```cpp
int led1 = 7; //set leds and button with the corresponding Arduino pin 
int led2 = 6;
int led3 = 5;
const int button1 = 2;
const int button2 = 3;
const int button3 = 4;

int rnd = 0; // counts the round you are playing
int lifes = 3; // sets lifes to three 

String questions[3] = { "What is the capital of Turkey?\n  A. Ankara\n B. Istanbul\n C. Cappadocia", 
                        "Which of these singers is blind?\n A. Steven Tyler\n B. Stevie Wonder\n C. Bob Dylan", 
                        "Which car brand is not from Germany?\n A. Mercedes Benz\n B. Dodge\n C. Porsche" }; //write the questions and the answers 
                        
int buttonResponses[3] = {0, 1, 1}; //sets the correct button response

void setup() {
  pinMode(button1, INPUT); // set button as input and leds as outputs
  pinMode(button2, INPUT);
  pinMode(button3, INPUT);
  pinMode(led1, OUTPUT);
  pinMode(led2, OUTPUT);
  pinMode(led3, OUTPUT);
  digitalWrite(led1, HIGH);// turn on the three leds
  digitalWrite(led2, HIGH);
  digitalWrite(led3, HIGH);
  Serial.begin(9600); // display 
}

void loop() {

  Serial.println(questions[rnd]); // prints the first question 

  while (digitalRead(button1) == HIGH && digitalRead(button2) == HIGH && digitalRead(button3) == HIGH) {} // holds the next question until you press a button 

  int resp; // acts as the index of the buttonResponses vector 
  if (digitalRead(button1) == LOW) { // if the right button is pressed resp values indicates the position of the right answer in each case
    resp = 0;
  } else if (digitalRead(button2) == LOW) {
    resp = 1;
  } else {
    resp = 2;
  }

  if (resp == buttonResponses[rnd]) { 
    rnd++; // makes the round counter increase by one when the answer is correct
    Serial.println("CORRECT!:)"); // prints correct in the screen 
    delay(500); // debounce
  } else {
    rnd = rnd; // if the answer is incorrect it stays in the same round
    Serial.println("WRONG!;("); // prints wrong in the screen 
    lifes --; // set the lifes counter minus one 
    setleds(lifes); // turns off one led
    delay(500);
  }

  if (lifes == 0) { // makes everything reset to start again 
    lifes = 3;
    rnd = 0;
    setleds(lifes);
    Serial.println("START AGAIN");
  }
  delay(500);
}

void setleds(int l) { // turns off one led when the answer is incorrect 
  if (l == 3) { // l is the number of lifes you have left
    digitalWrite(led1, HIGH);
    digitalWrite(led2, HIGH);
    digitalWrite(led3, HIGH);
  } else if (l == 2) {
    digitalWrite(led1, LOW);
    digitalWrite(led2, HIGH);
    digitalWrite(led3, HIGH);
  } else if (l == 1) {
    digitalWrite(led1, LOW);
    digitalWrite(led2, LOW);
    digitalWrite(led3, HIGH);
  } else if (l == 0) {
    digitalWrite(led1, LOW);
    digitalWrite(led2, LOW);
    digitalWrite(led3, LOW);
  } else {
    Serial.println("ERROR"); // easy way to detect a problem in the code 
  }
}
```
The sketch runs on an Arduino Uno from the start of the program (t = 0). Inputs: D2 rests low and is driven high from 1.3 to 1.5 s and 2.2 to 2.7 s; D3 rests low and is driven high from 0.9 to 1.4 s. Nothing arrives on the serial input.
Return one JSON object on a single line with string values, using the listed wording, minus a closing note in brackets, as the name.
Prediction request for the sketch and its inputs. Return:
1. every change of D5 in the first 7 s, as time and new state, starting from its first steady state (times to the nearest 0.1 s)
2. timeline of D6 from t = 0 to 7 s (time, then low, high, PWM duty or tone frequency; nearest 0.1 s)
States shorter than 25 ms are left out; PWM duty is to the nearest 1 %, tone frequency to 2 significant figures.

{"every change of D5 in the first 7 s, as time and new state, starting from its first steady state": "0 s high; 3.1 s low; 3.6 s high", "timeline of D6 from t = 0 to 7 s": "0 s high; 2.1 s low; 3.6 s high; 6.2 s low"}
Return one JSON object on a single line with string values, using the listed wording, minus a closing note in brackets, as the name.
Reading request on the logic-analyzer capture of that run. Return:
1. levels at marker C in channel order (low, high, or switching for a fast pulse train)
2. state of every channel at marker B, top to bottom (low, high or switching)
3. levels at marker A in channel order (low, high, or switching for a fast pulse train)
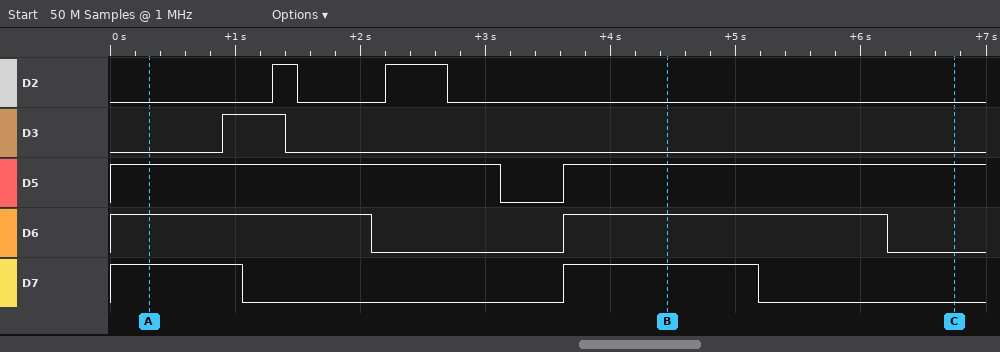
{"levels at marker C in channel order": "D2 low, D3 low, D5 high, D6 low, D7 low", "state of every channel at marker B, top to bottom": "D2 low, D3 low, D5 high, D6 high, D7 high", "levels at marker A in channel order": "D2 low, D3 low, D5 high, D6 high, D7 high"}
